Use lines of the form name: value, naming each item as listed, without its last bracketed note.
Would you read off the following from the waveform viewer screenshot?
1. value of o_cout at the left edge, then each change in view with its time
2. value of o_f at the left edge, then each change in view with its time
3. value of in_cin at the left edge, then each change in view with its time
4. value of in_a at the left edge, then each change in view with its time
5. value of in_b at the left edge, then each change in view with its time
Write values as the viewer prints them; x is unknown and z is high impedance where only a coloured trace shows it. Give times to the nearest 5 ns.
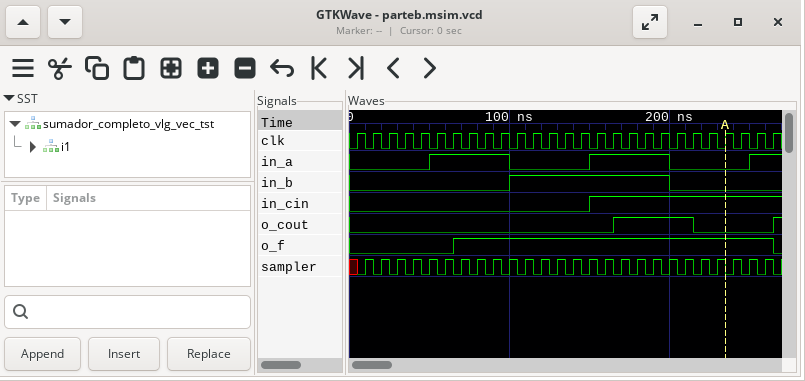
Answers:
value of o_cout at the left edge, then each change in view with its time: 0, 1 at 165 ns, 0 at 215 ns, 1 at 265 ns
value of o_f at the left edge, then each change in view with its time: 0, 1 at 65 ns, 0 at 265 ns
value of in_cin at the left edge, then each change in view with its time: 0, 1 at 150 ns
value of in_a at the left edge, then each change in view with its time: 0, 1 at 50 ns, 0 at 100 ns, 1 at 150 ns, 0 at 200 ns, 1 at 250 ns
value of in_b at the left edge, then each change in view with its time: 0, 1 at 100 ns, 0 at 200 ns
